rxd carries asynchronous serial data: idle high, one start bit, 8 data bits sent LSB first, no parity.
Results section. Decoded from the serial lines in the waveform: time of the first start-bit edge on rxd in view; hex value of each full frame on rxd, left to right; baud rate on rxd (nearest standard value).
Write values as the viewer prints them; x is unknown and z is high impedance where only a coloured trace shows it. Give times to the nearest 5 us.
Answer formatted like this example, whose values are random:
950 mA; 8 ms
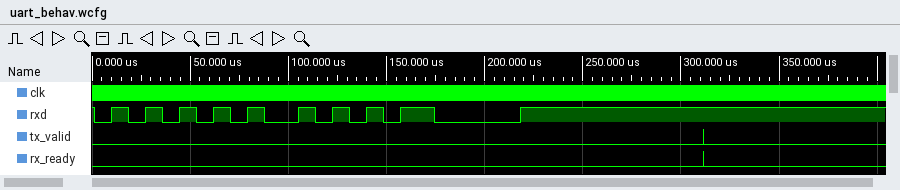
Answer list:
0 us; 55, AA, F0; 115200 baud
